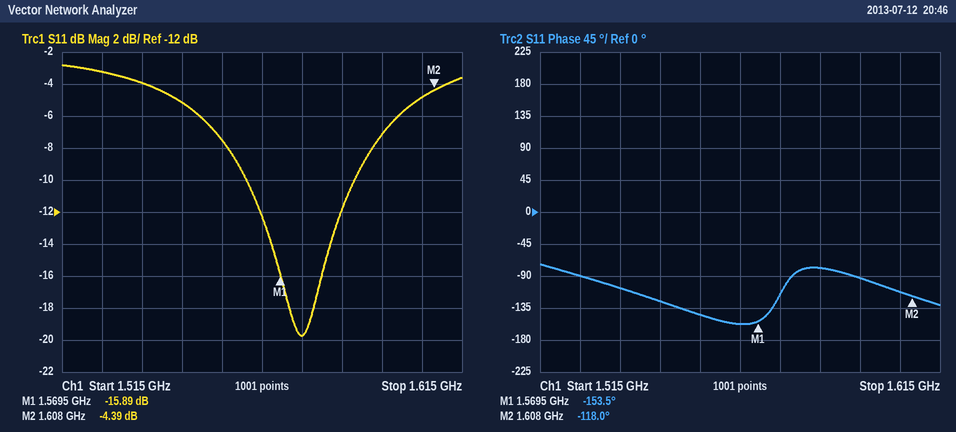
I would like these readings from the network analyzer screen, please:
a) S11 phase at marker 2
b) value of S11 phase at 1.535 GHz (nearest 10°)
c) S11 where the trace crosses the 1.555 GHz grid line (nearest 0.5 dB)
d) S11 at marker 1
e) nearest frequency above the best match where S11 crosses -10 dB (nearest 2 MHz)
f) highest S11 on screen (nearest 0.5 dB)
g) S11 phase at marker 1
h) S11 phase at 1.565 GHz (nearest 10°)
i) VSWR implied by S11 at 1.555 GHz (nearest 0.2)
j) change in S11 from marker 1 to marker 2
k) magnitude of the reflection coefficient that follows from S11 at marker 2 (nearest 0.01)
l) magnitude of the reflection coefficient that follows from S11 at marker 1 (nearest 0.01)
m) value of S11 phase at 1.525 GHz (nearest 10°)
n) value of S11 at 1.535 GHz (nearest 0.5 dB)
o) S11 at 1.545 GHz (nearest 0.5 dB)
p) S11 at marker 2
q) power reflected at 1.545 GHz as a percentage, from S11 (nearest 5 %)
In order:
-118.0°
-110°
-7.5 dB
-15.89 dB
1.588 GHz
-3.0 dB
-153.5°
-160°
2.4
11.50 dB
0.60
0.16
-90°
-4.0 dB
-5.0 dB
-4.39 dB
30 %
